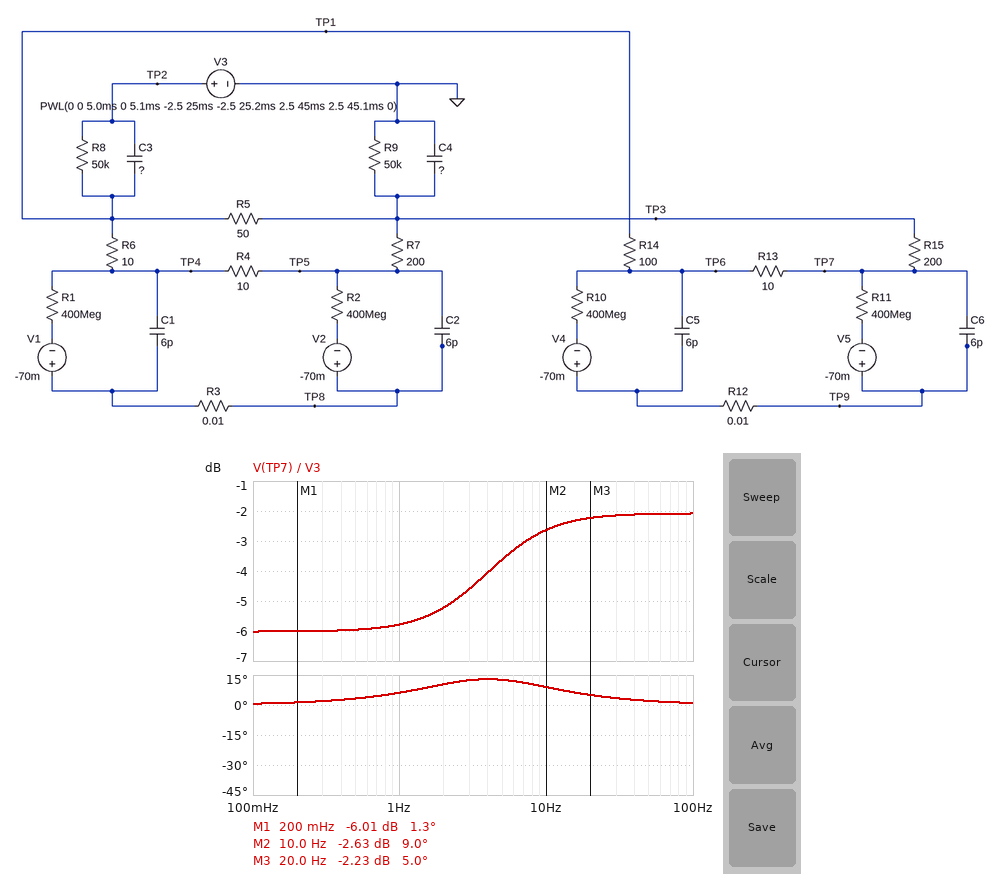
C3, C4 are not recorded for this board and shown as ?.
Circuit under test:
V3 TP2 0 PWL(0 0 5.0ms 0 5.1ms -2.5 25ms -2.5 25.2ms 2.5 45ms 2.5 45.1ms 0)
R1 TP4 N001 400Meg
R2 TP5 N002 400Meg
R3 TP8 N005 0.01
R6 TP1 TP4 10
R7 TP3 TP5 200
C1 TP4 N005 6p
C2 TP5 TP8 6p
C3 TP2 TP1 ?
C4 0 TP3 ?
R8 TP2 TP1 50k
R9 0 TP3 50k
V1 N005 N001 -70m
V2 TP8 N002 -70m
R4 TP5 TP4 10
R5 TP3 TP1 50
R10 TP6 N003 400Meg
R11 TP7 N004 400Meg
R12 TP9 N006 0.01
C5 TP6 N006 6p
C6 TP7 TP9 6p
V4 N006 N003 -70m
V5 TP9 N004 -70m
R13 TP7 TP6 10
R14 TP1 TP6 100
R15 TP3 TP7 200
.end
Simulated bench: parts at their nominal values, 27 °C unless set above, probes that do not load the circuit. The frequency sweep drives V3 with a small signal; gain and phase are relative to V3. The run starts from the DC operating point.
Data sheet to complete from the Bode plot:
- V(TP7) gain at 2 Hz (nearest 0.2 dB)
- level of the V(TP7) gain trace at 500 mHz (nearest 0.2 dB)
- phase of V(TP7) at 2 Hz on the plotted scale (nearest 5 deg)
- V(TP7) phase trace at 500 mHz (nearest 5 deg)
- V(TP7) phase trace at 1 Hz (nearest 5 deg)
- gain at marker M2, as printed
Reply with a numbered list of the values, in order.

1. -5.2 dB
2. -6.0 dB
3. 10 deg
4. 5 deg
5. 5 deg
6. -2.63 dB
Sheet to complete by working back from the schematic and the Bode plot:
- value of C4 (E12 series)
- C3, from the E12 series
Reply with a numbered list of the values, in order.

1. 270 nF
2. 1 µF
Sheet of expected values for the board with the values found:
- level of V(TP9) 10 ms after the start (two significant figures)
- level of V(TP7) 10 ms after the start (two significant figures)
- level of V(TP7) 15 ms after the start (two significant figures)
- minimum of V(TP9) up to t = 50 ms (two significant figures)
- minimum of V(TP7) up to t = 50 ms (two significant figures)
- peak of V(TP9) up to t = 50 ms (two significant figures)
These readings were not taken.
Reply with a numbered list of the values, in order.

1. -1.9 V
2. -1.9 V
3. -1.8 V
4. -2.0 V
5. -2.0 V
6. 2.2 V
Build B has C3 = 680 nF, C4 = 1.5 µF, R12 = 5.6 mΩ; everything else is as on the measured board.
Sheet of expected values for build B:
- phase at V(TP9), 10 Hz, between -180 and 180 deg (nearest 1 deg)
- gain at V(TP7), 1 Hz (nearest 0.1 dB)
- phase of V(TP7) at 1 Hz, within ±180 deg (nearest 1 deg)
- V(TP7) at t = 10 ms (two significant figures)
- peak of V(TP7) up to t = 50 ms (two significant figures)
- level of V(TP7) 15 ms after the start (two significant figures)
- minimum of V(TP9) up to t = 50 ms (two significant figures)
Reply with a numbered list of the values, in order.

1. -9 deg
2. -6.3 dB
3. -7 deg
4. -820 mV
5. 820 mV
6. -860 mV
7. -1.0 V
